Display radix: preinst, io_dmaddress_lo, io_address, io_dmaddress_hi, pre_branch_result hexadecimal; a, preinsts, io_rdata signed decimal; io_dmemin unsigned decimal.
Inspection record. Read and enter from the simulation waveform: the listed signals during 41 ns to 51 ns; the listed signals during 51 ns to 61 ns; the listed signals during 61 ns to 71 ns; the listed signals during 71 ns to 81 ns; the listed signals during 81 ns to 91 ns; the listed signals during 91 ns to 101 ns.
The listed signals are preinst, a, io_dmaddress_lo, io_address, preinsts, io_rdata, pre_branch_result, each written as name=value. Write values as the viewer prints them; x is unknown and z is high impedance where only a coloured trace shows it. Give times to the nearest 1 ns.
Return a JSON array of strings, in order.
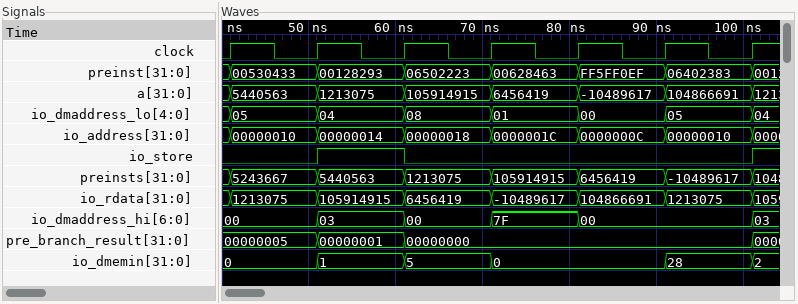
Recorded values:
["preinst=00530433, a=5440563, io_dmaddress_lo=05, io_address=00000010, preinsts=5243667, io_rdata=1213075, pre_branch_result=00000005", "preinst=00128293, a=1213075, io_dmaddress_lo=04, io_address=00000014, preinsts=5440563, io_rdata=105914915, pre_branch_result=00000001", "preinst=06502223, a=105914915, io_dmaddress_lo=08, io_address=00000018, preinsts=1213075, io_rdata=6456419, pre_branch_result=00000000", "preinst=00628463, a=6456419, io_dmaddress_lo=01, io_address=0000001C, preinsts=105914915, io_rdata=-10489617, pre_branch_result=00000000", "preinst=FF5FF0EF, a=-10489617, io_dmaddress_lo=00, io_address=0000000C, preinsts=6456419, io_rdata=104866691, pre_branch_result=00000000", "preinst=06402383, a=104866691, io_dmaddress_lo=05, io_address=00000010, preinsts=-10489617, io_rdata=1213075, pre_branch_result=00000000"]
